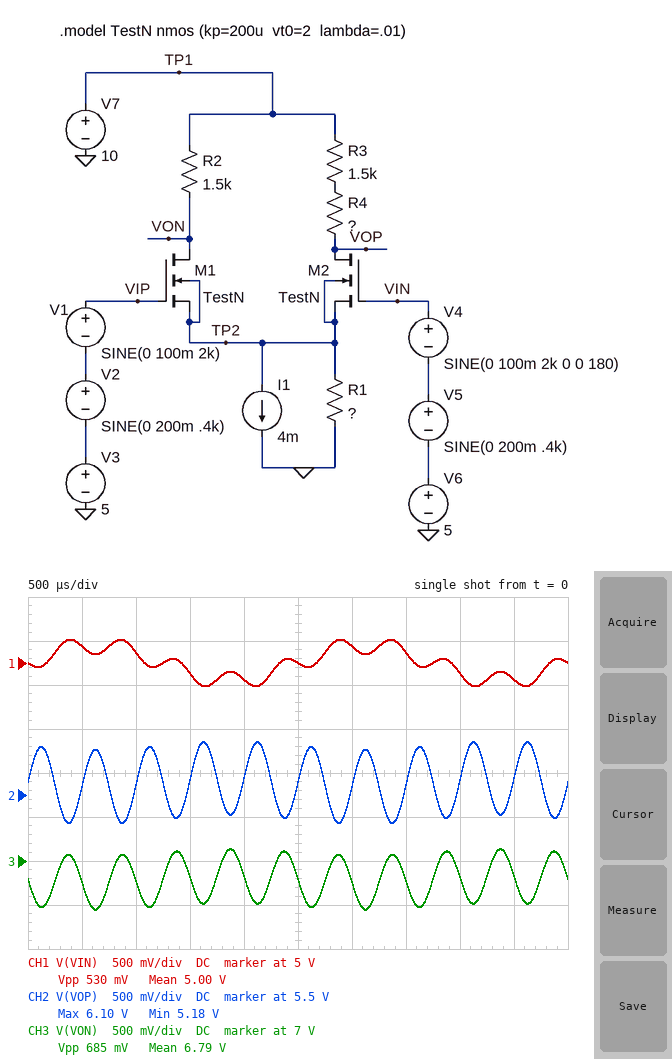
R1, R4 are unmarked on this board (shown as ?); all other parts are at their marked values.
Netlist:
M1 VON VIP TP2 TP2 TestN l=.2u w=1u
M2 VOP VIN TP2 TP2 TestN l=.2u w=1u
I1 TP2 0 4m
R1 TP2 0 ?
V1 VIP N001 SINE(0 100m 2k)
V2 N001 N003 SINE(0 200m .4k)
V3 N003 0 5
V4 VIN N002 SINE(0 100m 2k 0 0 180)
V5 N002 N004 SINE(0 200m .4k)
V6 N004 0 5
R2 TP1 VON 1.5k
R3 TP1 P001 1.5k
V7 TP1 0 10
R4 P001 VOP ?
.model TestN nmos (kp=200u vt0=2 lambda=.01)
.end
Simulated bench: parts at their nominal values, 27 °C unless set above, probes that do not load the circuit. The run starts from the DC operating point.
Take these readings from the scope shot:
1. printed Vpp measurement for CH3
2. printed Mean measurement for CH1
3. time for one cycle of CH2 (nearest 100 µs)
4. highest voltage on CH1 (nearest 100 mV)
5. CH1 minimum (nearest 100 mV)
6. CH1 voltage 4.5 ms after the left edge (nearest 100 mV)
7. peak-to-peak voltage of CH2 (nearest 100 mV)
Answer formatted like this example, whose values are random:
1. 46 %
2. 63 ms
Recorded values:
1. 685 mV
2. 5.00 V
3. 500 µs
4. 5.3 V
5. 4.7 V
6. 4.8 V
7. 900 mV
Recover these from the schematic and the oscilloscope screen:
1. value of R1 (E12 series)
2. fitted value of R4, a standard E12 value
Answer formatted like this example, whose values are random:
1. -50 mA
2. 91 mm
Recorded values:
1. 3.9 kΩ
2. 560 Ω
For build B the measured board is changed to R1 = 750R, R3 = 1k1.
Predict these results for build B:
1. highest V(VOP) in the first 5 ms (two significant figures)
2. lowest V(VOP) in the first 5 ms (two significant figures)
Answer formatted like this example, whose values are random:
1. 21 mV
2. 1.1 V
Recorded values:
1. 6.3 V
2. 5.3 V
